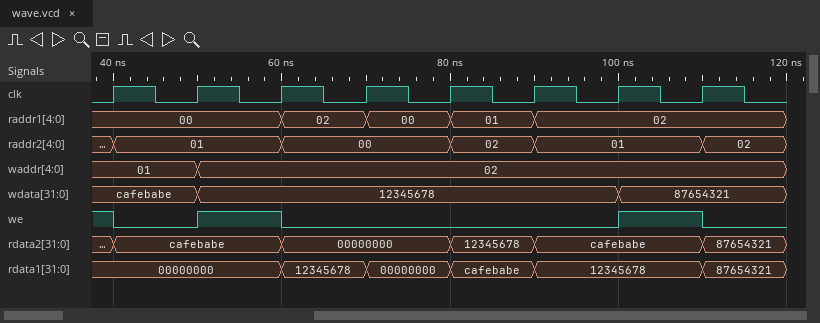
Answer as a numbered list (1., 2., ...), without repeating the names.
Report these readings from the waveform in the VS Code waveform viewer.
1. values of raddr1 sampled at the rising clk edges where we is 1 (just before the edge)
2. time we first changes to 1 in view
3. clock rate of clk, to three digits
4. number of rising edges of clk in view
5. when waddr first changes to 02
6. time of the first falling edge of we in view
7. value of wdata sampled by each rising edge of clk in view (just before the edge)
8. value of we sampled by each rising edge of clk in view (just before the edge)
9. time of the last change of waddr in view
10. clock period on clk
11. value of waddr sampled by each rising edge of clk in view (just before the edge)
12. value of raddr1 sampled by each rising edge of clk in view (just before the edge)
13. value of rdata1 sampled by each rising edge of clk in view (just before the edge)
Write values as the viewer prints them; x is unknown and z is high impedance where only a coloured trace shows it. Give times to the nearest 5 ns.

1. 00, 00, 02
2. 50 ns
3. 100 MHz
4. 8
5. 50 ns
6. 40 ns
7. cafebabe, cafebabe, 12345678, 12345678, 12345678, 12345678, 12345678, 87654321
8. 1 0 1 0 0 0 0 1
9. 50 ns
10. 10 ns
11. 01, 01, 02, 02, 02, 02, 02, 02
12. 00, 00, 00, 02, 00, 01, 02, 02
13. 00000000, 00000000, 00000000, 12345678, 00000000, cafebabe, 12345678, 12345678
